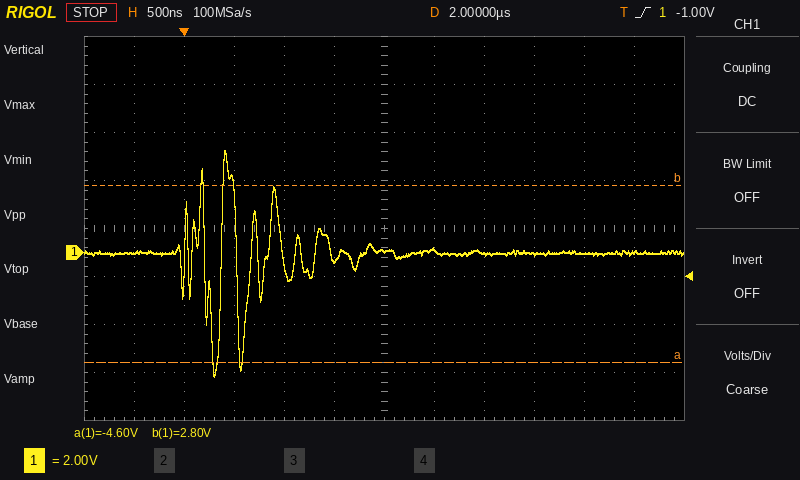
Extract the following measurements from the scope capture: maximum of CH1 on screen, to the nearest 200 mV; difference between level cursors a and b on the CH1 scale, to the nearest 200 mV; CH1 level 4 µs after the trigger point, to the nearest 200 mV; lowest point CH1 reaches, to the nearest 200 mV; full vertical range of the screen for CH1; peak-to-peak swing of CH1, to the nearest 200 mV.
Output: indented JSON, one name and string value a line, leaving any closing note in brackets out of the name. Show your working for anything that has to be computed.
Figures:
{
  "maximum of CH1 on screen, to the nearest 200 mV": "4.2 V",
  "difference between level cursors a and b on the CH1 scale, to the nearest 200 mV": "7.4 V",
  "CH1 level 4 µs after the trigger point, to the nearest 200 mV": "0.0 V",
  "lowest point CH1 reaches, to the nearest 200 mV": "-5.2 V",
  "full vertical range of the screen for CH1": "16 V",
  "peak-to-peak swing of CH1, to the nearest 200 mV": "4.2 V − (-5.2 V) = 9.4 V"
}
